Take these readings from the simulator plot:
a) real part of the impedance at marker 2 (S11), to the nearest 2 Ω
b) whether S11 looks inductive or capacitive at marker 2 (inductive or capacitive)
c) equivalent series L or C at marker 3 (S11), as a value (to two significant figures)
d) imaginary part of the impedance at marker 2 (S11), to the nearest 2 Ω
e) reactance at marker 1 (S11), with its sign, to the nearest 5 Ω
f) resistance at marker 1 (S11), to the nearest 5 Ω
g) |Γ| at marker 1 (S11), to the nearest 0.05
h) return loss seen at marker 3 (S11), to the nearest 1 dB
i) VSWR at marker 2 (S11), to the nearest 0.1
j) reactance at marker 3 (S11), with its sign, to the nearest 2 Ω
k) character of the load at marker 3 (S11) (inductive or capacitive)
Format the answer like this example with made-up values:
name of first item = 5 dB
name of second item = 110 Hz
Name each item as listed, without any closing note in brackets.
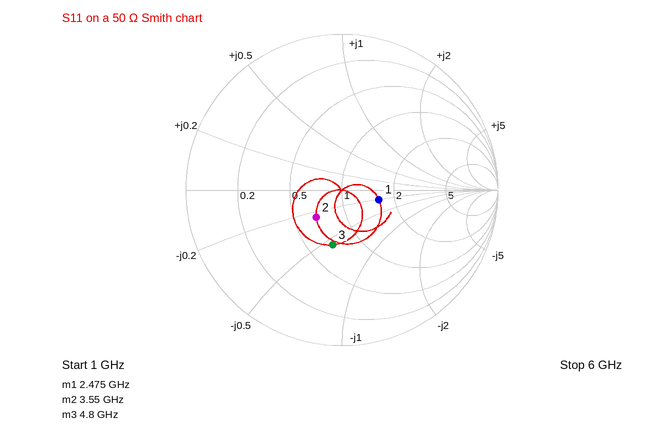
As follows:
real part of the impedance at marker 2 (S11), to the nearest 2 Ω = 34 Ω
whether S11 looks inductive or capacitive at marker 2 = capacitive
equivalent series L or C at marker 3 (S11), as a value = 1.2 pF
imaginary part of the impedance at marker 2 (S11), to the nearest 2 Ω = -12 Ω
reactance at marker 1 (S11), with its sign, to the nearest 5 Ω = -10 Ω
resistance at marker 1 (S11), to the nearest 5 Ω = 80 Ω
|Γ| at marker 1 (S11), to the nearest 0.05 = 0.25
return loss seen at marker 3 (S11), to the nearest 1 dB = 9 dB
VSWR at marker 2 (S11), to the nearest 0.1 = 1.6
reactance at marker 3 (S11), with its sign, to the nearest 2 Ω = -28 Ω
character of the load at marker 3 (S11) = capacitive
